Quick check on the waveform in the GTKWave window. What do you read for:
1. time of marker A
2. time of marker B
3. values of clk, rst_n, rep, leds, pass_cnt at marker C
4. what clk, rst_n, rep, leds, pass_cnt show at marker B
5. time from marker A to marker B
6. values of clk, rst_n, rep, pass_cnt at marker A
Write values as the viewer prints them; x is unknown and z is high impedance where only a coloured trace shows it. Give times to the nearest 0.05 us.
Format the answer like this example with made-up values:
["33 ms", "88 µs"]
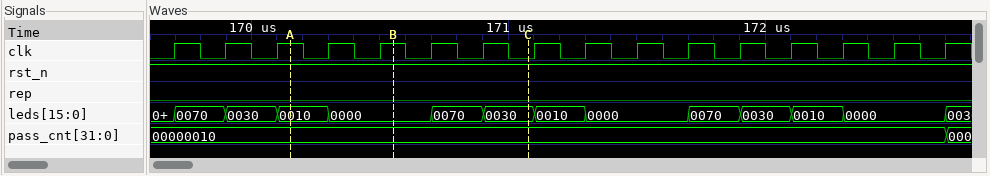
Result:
["170.15 us", "170.55 us", "clk=0, rst_n=1, rep=0, leds=0030, pass_cnt=00000010", "clk=1, rst_n=1, rep=0, leds=0000, pass_cnt=00000010", "0.4 us", "clk=1, rst_n=1, rep=0, pass_cnt=00000010"]
